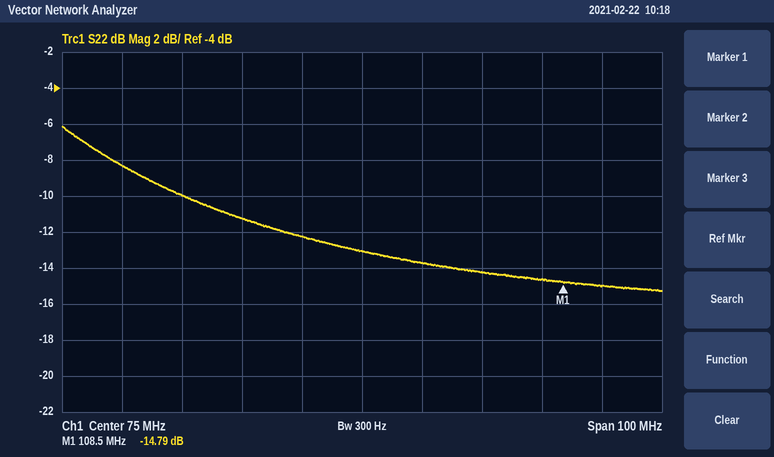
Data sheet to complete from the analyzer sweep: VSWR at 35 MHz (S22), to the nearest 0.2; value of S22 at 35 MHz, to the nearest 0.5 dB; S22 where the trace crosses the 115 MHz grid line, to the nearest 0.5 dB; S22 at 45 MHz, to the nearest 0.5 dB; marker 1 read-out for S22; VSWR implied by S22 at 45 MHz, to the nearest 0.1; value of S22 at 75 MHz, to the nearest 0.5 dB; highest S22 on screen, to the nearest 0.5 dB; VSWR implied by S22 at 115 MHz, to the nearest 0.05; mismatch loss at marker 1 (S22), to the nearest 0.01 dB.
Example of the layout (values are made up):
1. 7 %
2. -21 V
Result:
1. 2.2
2. -8.5 dB
3. -15.0 dB
4. -10.0 dB
5. -14.79 dB
6. 1.9
7. -13.0 dB
8. -6.0 dB
9. 1.45
10. 0.15 dB
